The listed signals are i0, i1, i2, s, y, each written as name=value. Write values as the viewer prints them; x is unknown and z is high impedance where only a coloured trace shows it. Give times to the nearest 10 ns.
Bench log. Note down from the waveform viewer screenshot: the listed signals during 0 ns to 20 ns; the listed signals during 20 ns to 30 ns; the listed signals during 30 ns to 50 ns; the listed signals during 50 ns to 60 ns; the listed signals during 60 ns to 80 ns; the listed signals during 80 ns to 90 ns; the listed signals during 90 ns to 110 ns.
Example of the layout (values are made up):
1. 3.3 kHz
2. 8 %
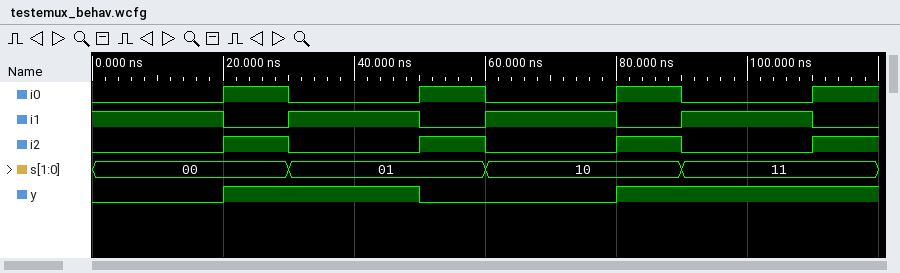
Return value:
1. i0=0, i1=1, i2=0, s=00, y=0
2. i0=1, i1=0, i2=1, s=00, y=1
3. i0=0, i1=1, i2=0, s=01, y=1
4. i0=1, i1=0, i2=1, s=01, y=0
5. i0=0, i1=1, i2=0, s=10, y=0
6. i0=1, i1=0, i2=1, s=10, y=1
7. i0=0, i1=1, i2=0, s=11, y=1
